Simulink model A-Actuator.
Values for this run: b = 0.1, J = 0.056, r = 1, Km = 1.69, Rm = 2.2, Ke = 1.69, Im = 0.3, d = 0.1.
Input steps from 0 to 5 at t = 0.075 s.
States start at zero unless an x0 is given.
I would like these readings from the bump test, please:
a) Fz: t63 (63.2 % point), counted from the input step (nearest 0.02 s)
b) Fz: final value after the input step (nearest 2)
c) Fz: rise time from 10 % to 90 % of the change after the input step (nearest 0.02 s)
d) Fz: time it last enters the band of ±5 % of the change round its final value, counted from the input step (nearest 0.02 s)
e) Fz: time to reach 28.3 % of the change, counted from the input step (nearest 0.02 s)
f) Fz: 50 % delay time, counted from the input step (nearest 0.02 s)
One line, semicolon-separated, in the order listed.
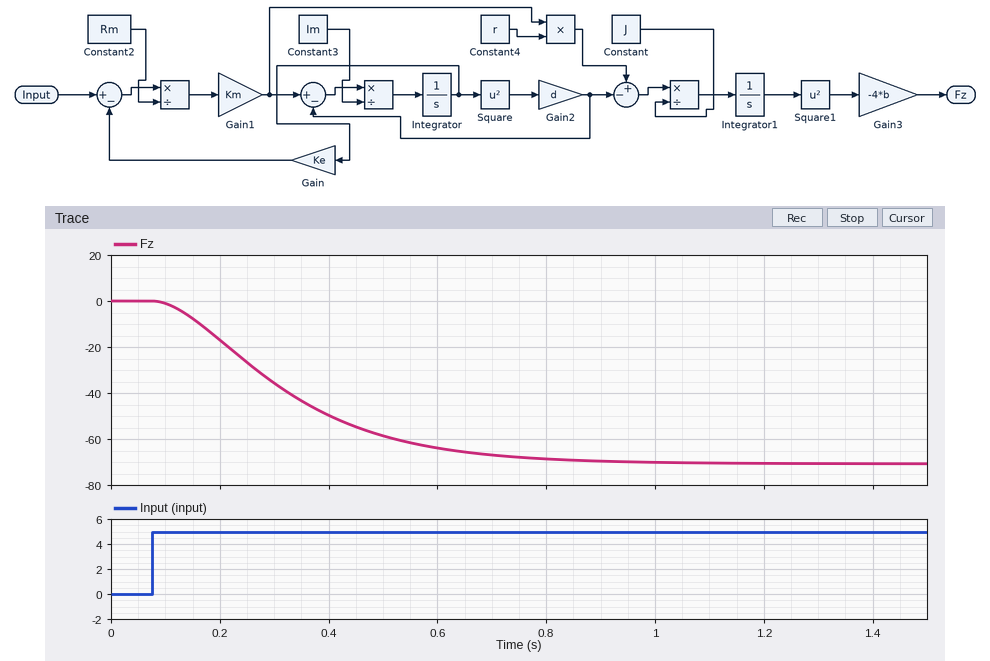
0.28 s; -70; 0.44 s; 0.64 s; 0.14 s; 0.22 s
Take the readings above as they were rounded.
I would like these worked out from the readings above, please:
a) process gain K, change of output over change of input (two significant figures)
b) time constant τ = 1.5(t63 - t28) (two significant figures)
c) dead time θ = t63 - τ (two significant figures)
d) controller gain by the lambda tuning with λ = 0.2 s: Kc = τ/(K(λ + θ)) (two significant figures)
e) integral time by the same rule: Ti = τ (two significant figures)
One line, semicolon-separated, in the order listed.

-14; 0.21 s; 0.070 s; -0.056; 0.21 s
